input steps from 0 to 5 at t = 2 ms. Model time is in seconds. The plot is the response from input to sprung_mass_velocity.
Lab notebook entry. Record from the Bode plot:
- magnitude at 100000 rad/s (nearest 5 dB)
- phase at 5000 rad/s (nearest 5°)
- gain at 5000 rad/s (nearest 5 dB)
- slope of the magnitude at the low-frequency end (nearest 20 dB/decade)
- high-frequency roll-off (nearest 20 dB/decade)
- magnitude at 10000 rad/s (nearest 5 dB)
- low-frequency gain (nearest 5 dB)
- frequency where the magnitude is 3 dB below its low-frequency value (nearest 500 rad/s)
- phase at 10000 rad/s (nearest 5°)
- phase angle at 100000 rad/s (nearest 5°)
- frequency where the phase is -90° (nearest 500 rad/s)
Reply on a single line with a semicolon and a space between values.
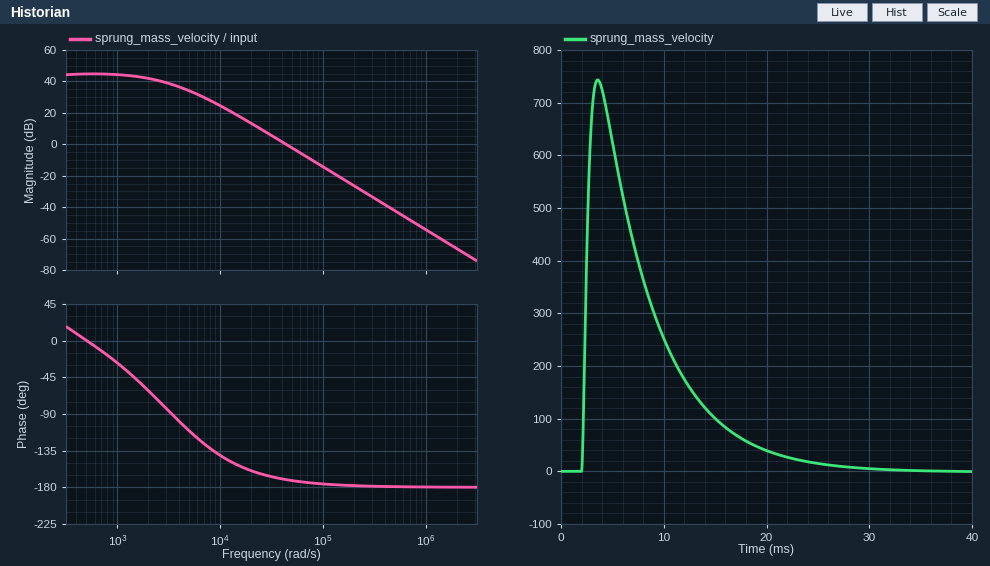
-15 dB; -110°; 35 dB; 0 dB/decade; -40 dB/decade; 25 dB; 45 dB; 2000 rad/s; -140°; -175°; 3500 rad/s
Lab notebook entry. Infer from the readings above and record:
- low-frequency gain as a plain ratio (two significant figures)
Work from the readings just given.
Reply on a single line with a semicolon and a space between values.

180
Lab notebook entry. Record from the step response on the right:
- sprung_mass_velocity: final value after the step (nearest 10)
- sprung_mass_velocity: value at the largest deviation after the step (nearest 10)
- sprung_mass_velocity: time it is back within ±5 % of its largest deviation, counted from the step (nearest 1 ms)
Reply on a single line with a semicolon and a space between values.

0; 740; 18 ms
